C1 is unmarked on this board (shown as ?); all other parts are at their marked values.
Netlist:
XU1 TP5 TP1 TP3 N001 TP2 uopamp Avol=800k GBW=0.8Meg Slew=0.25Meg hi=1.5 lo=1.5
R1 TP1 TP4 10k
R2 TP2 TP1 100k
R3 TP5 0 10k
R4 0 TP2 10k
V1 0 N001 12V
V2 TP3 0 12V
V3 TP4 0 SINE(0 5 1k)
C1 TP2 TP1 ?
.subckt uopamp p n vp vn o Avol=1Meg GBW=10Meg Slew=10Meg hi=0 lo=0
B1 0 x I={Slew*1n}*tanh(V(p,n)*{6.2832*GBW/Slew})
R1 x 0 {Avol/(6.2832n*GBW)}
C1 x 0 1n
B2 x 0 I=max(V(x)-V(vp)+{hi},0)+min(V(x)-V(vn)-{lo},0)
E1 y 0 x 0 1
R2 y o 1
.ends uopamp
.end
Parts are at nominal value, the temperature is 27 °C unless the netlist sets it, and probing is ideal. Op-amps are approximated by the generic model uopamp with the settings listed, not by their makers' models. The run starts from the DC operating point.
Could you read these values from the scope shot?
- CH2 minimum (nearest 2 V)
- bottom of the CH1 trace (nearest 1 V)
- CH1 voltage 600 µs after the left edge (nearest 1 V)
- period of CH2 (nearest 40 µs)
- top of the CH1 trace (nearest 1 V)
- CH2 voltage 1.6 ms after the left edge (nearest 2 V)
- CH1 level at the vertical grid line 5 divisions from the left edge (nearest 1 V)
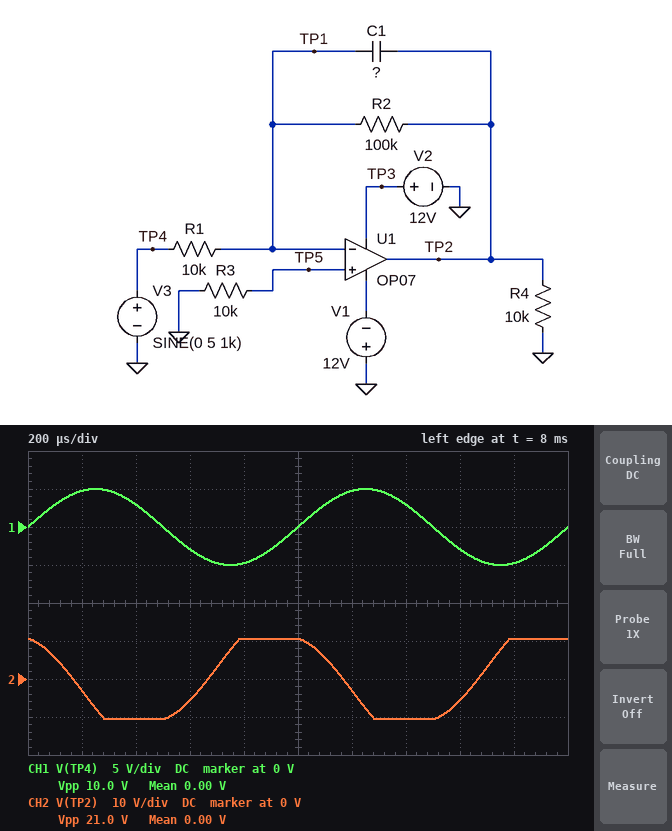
-10 V
-5 V
-3 V
1.00 ms
5 V
-6 V
0 V
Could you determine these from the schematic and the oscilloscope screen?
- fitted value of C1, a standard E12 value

4.7 nF
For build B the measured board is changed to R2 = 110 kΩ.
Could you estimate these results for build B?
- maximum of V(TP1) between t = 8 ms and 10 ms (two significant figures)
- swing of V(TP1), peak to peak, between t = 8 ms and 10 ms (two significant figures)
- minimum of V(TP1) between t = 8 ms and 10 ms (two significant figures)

2.6 V
5.1 V
-2.6 V
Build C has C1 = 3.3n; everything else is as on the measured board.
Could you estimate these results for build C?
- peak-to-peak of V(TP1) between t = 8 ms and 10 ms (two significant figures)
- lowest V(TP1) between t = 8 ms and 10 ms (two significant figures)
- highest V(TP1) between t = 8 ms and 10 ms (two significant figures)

6.5 V
-3.3 V
3.3 V
